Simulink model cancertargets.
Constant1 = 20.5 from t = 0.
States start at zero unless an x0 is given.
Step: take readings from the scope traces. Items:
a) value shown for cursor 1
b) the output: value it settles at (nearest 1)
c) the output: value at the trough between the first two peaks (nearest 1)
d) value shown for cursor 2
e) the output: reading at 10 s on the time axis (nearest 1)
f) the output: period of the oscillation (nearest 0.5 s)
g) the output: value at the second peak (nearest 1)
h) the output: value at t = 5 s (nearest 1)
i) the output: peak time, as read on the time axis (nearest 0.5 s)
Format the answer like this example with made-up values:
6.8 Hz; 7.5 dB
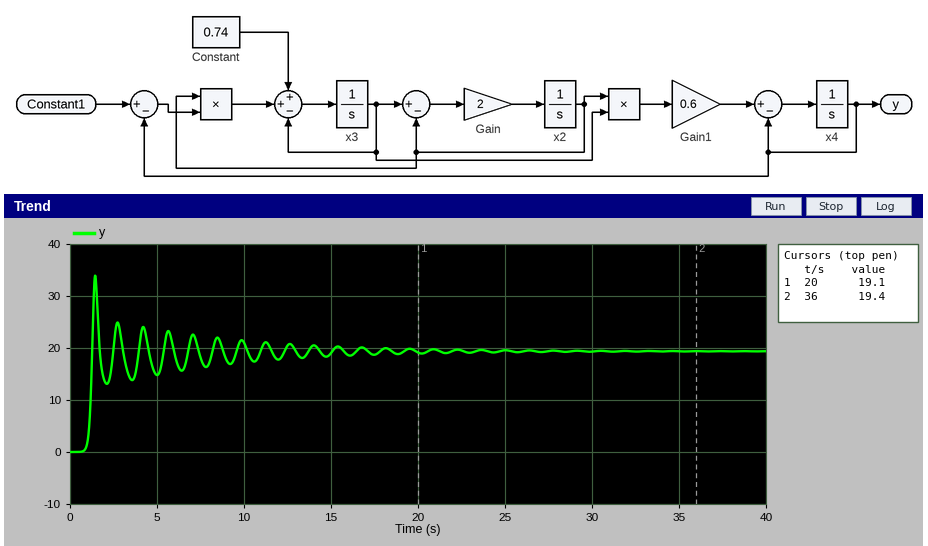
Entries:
19.1; 19; 13; 19.4; 21; 1.5 s; 25; 15; 1.5 s
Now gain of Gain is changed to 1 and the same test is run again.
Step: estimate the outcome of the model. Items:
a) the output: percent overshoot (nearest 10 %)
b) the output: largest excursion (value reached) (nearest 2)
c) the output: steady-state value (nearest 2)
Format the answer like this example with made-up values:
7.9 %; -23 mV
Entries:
60 %; 32; 20
